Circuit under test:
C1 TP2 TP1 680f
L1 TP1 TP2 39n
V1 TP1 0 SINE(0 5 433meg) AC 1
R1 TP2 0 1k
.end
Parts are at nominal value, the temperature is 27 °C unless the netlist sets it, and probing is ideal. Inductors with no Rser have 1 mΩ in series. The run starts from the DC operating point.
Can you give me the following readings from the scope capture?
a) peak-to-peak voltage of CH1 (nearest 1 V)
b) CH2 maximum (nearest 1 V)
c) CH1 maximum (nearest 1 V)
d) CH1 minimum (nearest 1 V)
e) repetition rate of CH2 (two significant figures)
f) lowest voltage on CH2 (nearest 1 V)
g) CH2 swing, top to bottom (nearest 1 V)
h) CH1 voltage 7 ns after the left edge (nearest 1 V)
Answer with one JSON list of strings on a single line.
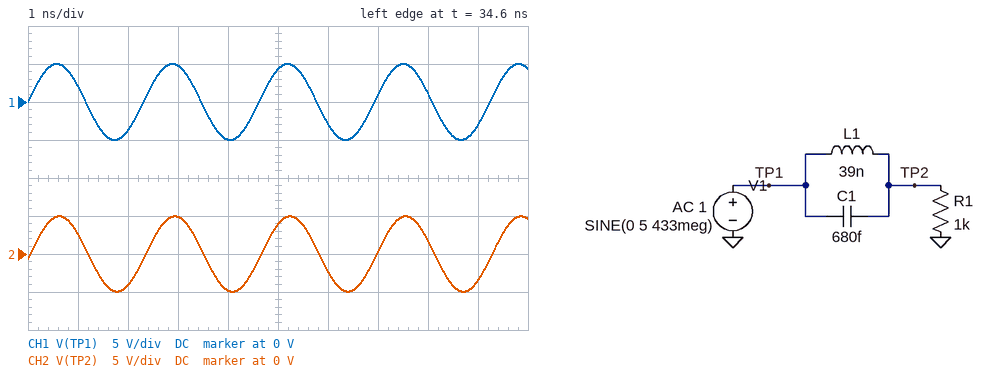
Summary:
["10 V", "5 V", "5 V", "-5 V", "430 MHz", "-5 V", "10 V", "1 V"]
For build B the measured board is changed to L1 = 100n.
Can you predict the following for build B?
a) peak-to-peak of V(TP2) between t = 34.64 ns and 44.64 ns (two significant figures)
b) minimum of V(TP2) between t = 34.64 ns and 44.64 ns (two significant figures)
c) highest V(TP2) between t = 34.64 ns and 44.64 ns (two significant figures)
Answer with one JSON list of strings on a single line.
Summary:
["8.8 V", "-4.4 V", "4.4 V"]
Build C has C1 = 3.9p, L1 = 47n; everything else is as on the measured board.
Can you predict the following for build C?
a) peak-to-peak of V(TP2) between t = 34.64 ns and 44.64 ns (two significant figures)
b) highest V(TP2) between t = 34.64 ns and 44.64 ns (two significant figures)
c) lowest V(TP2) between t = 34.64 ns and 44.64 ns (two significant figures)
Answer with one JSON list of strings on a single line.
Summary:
["9.4 V", "4.7 V", "-4.7 V"]
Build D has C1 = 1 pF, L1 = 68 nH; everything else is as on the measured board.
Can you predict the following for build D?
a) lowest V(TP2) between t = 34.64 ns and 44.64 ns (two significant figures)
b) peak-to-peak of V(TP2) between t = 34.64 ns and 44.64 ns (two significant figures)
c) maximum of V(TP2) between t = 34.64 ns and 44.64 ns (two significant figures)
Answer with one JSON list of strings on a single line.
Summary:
["-4.7 V", "9.4 V", "4.7 V"]
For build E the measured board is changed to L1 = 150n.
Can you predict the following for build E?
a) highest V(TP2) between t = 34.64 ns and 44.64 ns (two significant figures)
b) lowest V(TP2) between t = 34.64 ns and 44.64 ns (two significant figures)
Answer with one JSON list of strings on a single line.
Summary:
["2.6 V", "-2.6 V"]
